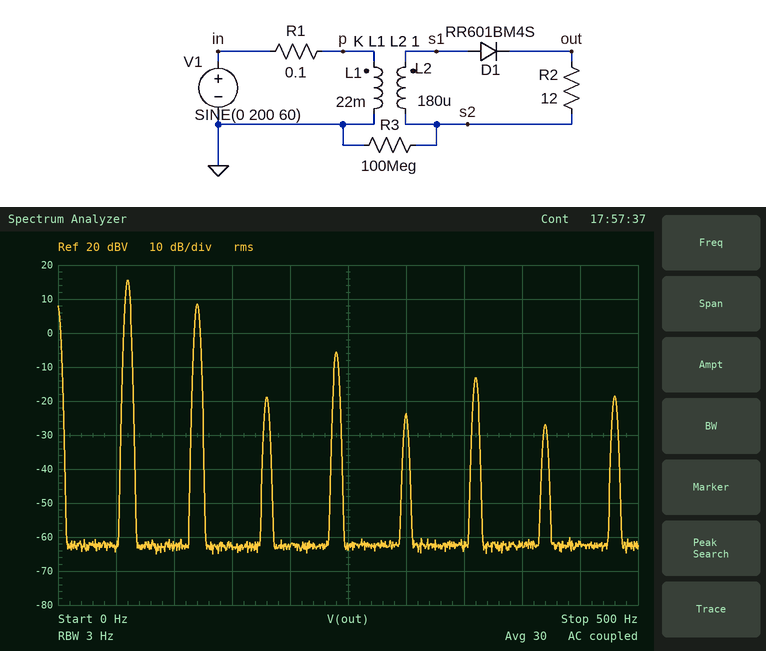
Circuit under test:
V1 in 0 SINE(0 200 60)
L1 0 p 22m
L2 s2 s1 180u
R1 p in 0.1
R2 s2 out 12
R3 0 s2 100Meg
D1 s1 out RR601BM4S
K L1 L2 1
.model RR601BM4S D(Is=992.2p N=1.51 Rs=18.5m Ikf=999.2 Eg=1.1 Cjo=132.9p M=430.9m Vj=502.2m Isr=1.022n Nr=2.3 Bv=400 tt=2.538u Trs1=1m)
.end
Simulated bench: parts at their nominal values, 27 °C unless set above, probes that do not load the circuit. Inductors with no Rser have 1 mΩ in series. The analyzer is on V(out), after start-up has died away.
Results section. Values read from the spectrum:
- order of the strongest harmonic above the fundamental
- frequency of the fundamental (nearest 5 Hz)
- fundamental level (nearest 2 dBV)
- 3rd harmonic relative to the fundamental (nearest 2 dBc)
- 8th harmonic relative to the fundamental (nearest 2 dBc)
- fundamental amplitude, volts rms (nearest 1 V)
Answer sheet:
2
60 Hz
16 dBV
-34 dBc
-34 dBc
6 V
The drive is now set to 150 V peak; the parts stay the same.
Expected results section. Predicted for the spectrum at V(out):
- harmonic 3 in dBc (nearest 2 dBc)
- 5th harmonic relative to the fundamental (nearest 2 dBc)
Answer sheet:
-32 dBc
-36 dBc
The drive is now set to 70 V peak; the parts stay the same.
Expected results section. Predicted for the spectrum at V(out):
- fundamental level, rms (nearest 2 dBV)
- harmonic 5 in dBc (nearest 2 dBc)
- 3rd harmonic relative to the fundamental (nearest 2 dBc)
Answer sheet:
6 dBV
-30 dBc
-26 dBc
